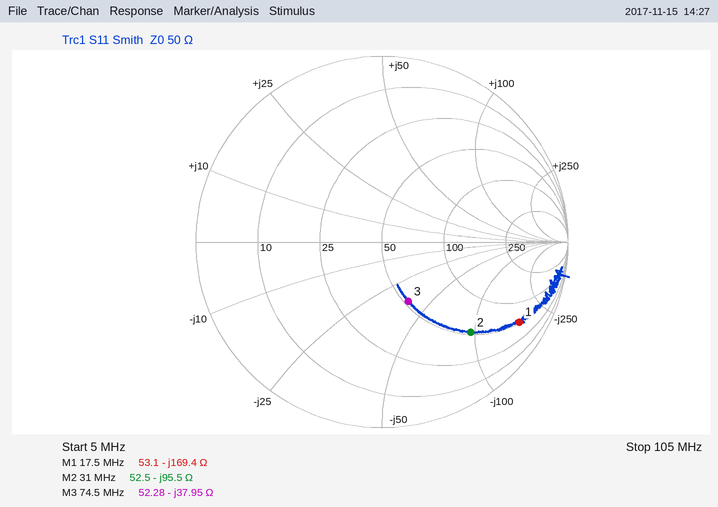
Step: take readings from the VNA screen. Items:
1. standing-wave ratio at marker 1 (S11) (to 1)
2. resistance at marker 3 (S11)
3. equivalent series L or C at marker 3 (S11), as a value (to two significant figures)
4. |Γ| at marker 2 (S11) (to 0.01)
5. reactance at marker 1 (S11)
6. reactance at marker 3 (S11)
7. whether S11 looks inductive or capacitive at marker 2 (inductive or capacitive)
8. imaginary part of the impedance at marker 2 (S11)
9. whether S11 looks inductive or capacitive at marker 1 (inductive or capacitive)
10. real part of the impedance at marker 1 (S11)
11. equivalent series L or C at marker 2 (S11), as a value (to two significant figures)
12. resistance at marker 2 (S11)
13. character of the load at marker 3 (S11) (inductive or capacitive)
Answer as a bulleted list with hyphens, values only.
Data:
- 13
- 52.28 Ω
- 56 pF
- 0.68
- -169.4 Ω
- -37.95 Ω
- capacitive
- -95.5 Ω
- capacitive
- 53.1 Ω
- 54 pF
- 52.5 Ω
- capacitive
